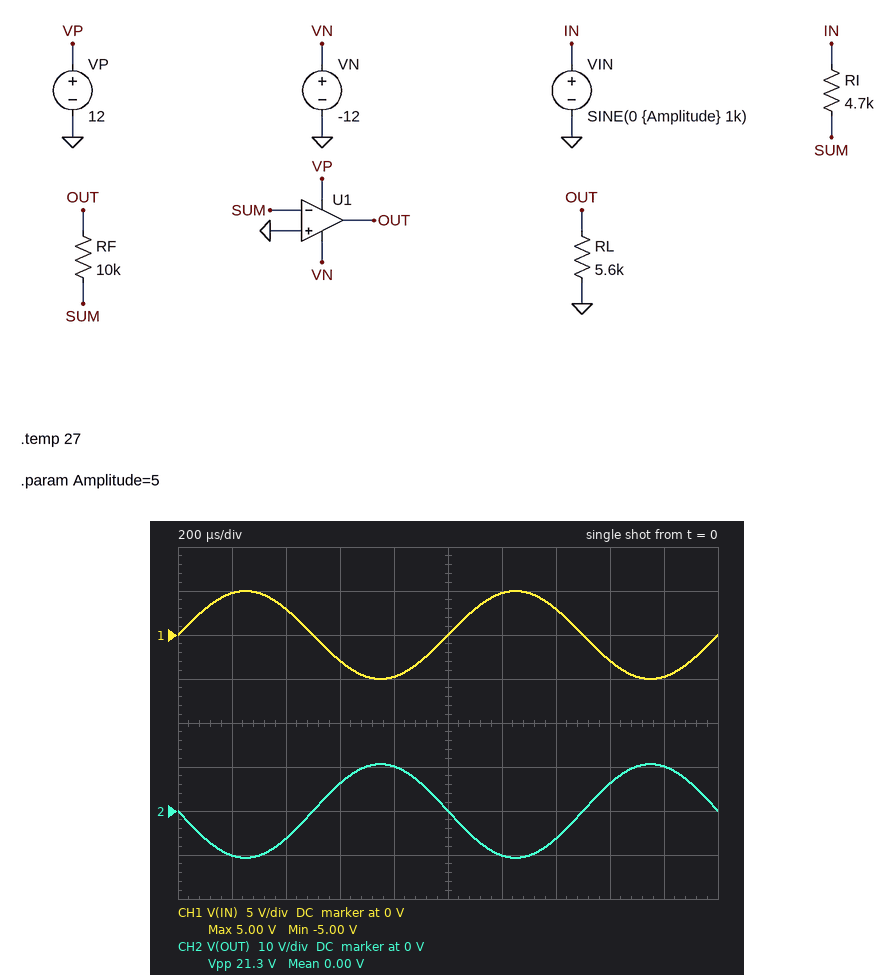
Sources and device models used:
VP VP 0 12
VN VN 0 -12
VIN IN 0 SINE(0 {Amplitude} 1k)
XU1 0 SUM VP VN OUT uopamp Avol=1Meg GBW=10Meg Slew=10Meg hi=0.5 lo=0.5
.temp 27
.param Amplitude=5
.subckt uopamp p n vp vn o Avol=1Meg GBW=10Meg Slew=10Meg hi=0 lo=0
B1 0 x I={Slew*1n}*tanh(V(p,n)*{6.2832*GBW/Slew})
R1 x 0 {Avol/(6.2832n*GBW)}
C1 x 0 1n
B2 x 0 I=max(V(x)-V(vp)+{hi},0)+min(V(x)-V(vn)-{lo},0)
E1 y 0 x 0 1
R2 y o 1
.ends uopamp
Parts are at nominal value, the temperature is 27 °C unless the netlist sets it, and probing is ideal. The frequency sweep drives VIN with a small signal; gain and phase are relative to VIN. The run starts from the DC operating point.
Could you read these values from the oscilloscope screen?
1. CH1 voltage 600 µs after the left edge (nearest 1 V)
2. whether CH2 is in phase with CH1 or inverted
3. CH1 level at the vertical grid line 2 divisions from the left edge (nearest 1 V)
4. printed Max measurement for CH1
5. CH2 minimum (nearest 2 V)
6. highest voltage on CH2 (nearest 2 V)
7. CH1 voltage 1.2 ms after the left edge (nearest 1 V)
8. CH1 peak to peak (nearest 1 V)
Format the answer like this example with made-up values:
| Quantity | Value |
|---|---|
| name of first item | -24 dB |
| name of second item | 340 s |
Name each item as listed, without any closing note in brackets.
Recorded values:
| Quantity | Value |
|---|---|
| CH1 voltage 600 µs after the left edge | -3 V |
| whether CH2 is in phase with CH1 or inverted | inverted |
| CH1 level at the vertical grid line 2 divisions from the left edge | 3 V |
| printed Max measurement for CH1 | 5.00 V |
| CH2 minimum | -10 V |
| highest voltage on CH2 | 10 V |
| CH1 voltage 1.2 ms after the left edge | 5 V |
| CH1 peak to peak | 10 V |
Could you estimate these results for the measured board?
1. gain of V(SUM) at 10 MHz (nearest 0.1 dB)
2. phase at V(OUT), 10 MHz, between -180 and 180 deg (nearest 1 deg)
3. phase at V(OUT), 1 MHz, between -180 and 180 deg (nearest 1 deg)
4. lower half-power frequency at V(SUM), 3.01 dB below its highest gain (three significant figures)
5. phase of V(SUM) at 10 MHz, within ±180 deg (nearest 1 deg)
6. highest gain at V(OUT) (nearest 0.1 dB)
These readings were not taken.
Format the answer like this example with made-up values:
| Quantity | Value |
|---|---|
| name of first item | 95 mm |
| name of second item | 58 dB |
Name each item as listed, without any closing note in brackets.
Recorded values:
| Quantity | Value |
|---|---|
| gain of V(SUM) at 10 MHz | -3.8 dB |
| phase at V(OUT), 10 MHz, between -180 and 180 deg | 108 deg |
| phase at V(OUT), 1 MHz, between -180 and 180 deg | 163 deg |
| lower half-power frequency at V(SUM), 3.01 dB below its highest gain | 3.20 MHz |
| phase of V(SUM) at 10 MHz, within ±180 deg | 18 deg |
| highest gain at V(OUT) | 6.6 dB |
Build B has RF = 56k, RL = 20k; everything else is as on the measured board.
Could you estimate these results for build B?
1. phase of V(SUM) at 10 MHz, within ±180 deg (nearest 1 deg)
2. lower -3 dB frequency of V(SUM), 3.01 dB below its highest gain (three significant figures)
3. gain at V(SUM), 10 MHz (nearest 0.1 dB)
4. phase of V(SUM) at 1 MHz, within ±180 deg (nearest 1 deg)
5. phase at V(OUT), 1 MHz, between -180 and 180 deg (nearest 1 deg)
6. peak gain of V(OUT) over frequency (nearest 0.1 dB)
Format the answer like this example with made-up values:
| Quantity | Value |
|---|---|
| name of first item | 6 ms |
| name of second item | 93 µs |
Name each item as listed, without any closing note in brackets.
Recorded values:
| Quantity | Value |
|---|---|
| phase of V(SUM) at 10 MHz, within ±180 deg | 4 deg |
| lower -3 dB frequency of V(SUM), 3.01 dB below its highest gain | 774 kHz |
| gain at V(SUM), 10 MHz | -0.7 dB |
| phase of V(SUM) at 1 MHz, within ±180 deg | 38 deg |
| phase at V(OUT), 1 MHz, between -180 and 180 deg | 128 deg |
| peak gain of V(OUT) over frequency | 21.5 dB |
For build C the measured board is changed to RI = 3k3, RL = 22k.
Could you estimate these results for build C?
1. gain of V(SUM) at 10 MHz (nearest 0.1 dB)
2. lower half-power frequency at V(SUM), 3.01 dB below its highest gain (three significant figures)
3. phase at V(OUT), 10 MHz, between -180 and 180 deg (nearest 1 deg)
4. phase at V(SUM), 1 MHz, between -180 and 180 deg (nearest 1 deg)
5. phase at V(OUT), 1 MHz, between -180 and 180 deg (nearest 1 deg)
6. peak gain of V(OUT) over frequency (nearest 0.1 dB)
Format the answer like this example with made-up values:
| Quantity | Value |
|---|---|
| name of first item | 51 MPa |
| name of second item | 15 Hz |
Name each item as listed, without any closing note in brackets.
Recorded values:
| Quantity | Value |
|---|---|
| gain of V(SUM) at 10 MHz | -2.7 dB |
| lower half-power frequency at V(SUM), 3.01 dB below its highest gain | 2.48 MHz |
| phase at V(OUT), 10 MHz, between -180 and 180 deg | 104 deg |
| phase at V(SUM), 1 MHz, between -180 and 180 deg | 68 deg |
| phase at V(OUT), 1 MHz, between -180 and 180 deg | 158 deg |
| peak gain of V(OUT) over frequency | 9.6 dB |
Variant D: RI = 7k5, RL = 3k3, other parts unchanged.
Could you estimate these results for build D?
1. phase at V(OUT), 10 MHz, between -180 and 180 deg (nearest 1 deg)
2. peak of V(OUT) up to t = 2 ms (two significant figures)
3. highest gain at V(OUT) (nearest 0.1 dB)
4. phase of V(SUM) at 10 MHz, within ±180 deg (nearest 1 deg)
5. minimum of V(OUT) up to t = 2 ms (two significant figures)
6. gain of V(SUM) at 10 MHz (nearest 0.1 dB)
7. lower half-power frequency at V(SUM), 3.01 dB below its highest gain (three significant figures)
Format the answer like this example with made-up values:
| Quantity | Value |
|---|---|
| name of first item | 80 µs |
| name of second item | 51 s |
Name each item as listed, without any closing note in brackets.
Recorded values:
| Quantity | Value |
|---|---|
| phase at V(OUT), 10 MHz, between -180 and 180 deg | 113 deg |
| peak of V(OUT) up to t = 2 ms | 6.7 V |
| highest gain at V(OUT) | 2.5 dB |
| phase of V(SUM) at 10 MHz, within ±180 deg | 23 deg |
| minimum of V(OUT) up to t = 2 ms | -6.7 V |
| gain of V(SUM) at 10 MHz | -5.6 dB |
| lower half-power frequency at V(SUM), 3.01 dB below its highest gain | 4.28 MHz |
